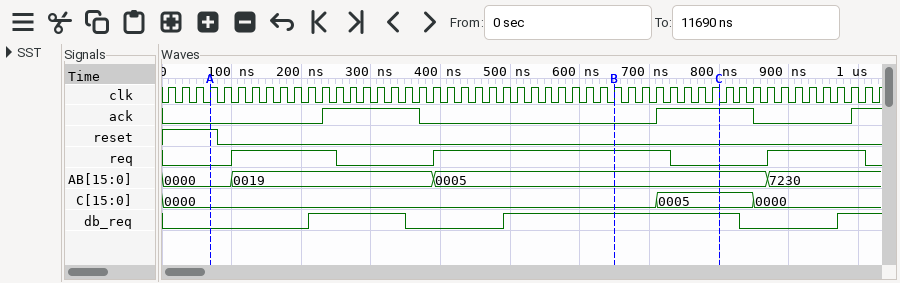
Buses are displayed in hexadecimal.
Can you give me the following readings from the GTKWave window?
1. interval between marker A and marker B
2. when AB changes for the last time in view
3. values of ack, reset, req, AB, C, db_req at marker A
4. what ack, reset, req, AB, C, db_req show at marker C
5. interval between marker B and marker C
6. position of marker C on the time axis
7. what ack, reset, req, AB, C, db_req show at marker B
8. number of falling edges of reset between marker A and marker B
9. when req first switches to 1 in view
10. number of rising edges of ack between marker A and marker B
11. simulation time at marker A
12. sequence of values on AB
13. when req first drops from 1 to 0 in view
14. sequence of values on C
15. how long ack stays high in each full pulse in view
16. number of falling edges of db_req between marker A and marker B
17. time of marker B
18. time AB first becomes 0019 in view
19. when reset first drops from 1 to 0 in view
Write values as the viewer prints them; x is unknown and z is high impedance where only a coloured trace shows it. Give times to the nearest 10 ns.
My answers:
580 ns
870 ns
ack=0, reset=1, req=0, AB=0000, C=0000, db_req=0
ack=1, reset=0, req=0, AB=0005, C=0005, db_req=1
150 ns
800 ns
ack=0, reset=0, req=1, AB=0005, C=0000, db_req=1
1
100 ns
1
70 ns
0000, 0019, 0005, 7230
250 ns
0000, 0005, 0000
140 ns, 140 ns
1
650 ns
100 ns
80 ns
